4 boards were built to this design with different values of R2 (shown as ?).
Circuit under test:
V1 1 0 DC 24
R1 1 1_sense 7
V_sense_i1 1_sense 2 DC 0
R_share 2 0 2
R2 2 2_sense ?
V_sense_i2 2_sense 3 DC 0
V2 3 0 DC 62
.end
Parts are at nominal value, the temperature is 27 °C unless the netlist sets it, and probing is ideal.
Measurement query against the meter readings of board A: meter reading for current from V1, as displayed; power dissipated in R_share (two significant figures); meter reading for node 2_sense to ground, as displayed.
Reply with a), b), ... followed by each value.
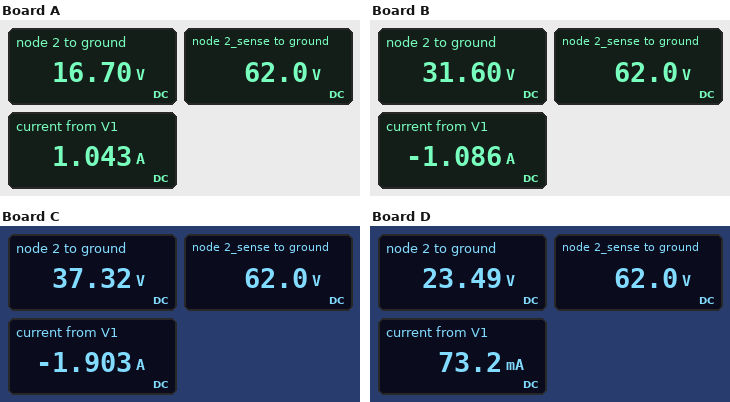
a) 1.043 A
b) 140 W
c) 62.0 V
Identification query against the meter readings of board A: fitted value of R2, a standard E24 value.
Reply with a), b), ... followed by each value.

a) 6.2 Ω
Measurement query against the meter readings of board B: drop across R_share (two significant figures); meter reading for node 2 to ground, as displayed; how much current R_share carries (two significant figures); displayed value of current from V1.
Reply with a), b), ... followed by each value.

a) 32 V
b) 31.60 V
c) 16 A
d) -1.086 A
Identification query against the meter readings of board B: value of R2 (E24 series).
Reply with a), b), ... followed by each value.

a) 1.8 Ω
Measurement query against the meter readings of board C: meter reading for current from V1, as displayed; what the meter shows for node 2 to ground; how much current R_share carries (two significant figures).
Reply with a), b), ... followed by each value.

a) -1.903 A
b) 37.32 V
c) 19 A
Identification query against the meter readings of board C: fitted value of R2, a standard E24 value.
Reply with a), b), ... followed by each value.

a) 1.2 Ω
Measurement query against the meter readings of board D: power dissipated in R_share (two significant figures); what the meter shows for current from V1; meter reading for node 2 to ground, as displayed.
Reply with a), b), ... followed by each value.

a) 280 W
b) 73.2 mA
c) 23.49 V
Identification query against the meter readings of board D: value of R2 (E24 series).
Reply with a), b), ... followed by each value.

a) 3.3 Ω
